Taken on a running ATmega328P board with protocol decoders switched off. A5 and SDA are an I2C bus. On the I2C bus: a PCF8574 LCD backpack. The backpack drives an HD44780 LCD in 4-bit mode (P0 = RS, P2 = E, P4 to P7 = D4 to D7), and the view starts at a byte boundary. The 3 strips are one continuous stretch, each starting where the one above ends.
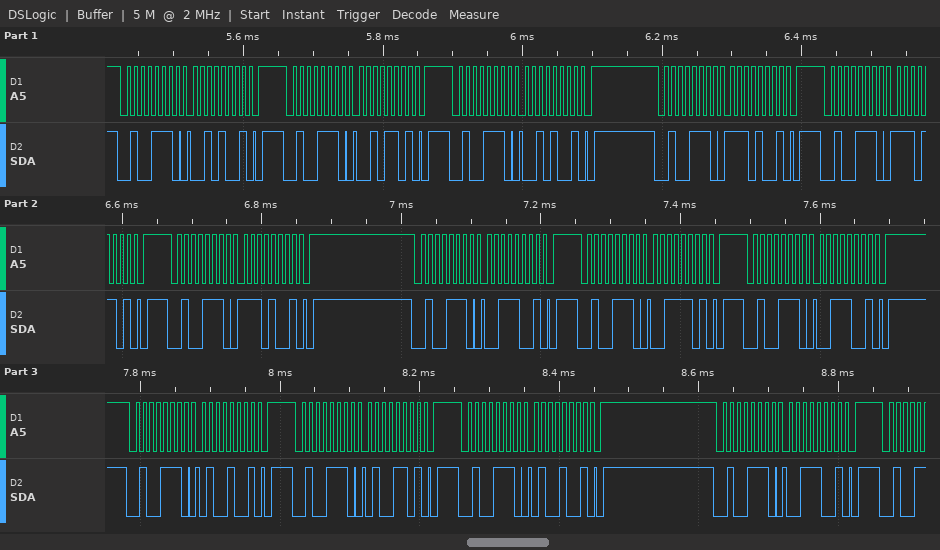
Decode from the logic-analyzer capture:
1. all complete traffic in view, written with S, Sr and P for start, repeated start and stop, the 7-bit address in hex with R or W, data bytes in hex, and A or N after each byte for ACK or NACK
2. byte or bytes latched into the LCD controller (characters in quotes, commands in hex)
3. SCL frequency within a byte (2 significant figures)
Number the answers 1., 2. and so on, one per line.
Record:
1. S 27W A 29 A P S 27W A 2D A P S 27W A 29 A P S 27W A E9 A P S 27W A ED A P S 27W A E9 A P S 27W A 39 A P S 27W A 3D A P S 27W A 39 A P S 27W A 49 A P S 27W A 4D A P S 27W A 49 A P S 27W A 39 A P
2. '.' '4'
3. 100 kHz
